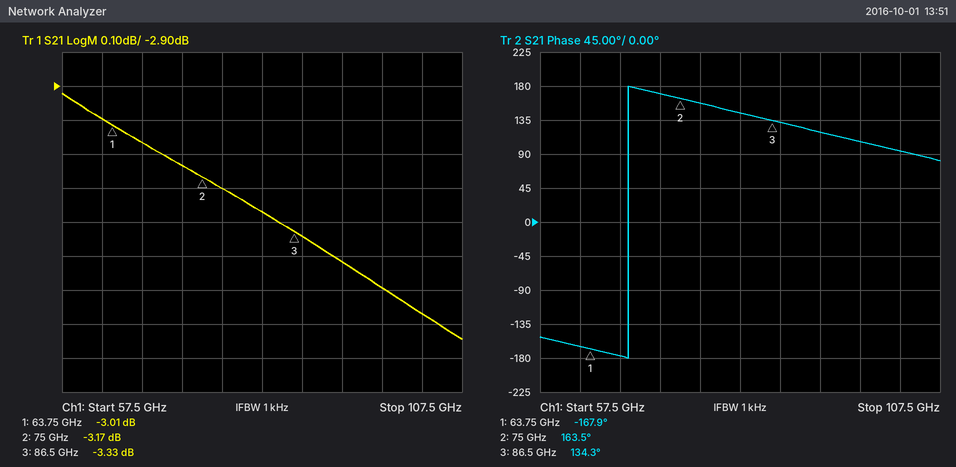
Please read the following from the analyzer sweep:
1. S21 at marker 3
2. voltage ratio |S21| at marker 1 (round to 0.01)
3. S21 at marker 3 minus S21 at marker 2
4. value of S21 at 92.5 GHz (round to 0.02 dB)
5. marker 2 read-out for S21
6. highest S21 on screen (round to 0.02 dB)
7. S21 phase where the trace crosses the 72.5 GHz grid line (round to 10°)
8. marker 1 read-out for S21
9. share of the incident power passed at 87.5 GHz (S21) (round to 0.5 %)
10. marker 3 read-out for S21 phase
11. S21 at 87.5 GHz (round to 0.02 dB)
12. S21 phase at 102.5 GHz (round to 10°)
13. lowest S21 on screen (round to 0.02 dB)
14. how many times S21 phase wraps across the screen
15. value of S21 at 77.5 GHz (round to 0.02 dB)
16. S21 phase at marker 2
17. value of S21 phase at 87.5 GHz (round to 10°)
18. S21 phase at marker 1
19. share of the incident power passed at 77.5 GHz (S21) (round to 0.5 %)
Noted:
-3.33 dB
0.71
-0.16 dB
-3.42 dB
-3.17 dB
-2.92 dB
170°
-3.01 dB
46.5 %
134.3°
-3.34 dB
90°
-3.64 dB
1
-3.20 dB
163.5°
130°
-167.9°
48.0 %
